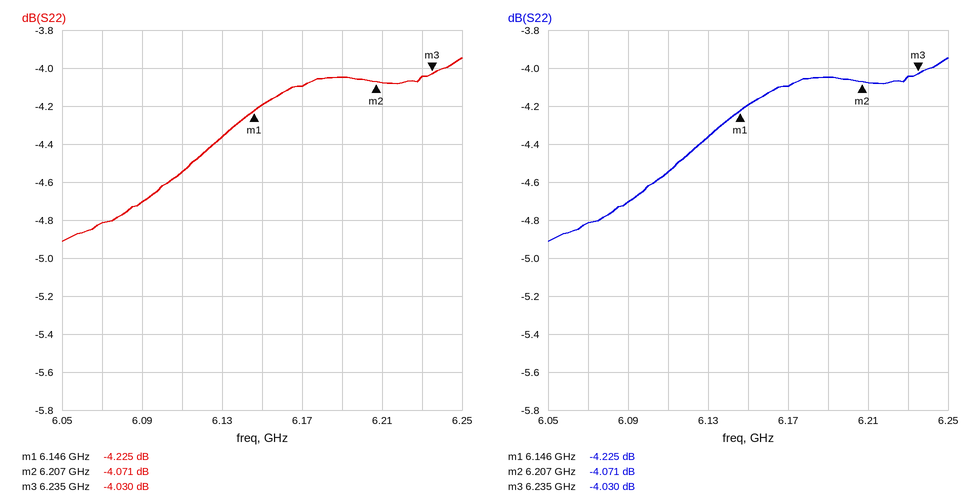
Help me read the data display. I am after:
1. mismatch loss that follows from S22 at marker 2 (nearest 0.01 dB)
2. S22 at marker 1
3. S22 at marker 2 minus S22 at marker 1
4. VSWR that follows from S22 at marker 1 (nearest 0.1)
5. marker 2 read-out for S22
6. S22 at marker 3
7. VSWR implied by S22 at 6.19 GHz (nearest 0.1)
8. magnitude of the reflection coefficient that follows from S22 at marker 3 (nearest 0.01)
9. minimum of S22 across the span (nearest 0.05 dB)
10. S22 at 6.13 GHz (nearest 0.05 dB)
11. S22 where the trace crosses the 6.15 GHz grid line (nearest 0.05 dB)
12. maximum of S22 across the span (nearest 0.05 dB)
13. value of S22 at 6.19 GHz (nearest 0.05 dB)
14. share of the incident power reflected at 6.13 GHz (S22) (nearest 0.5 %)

2.16 dB
-4.225 dB
0.154 dB
4.2
-4.071 dB
-4.030 dB
4.4
0.63
-4.90 dB
-4.35 dB
-4.20 dB
-3.95 dB
-4.05 dB
36.5 %
